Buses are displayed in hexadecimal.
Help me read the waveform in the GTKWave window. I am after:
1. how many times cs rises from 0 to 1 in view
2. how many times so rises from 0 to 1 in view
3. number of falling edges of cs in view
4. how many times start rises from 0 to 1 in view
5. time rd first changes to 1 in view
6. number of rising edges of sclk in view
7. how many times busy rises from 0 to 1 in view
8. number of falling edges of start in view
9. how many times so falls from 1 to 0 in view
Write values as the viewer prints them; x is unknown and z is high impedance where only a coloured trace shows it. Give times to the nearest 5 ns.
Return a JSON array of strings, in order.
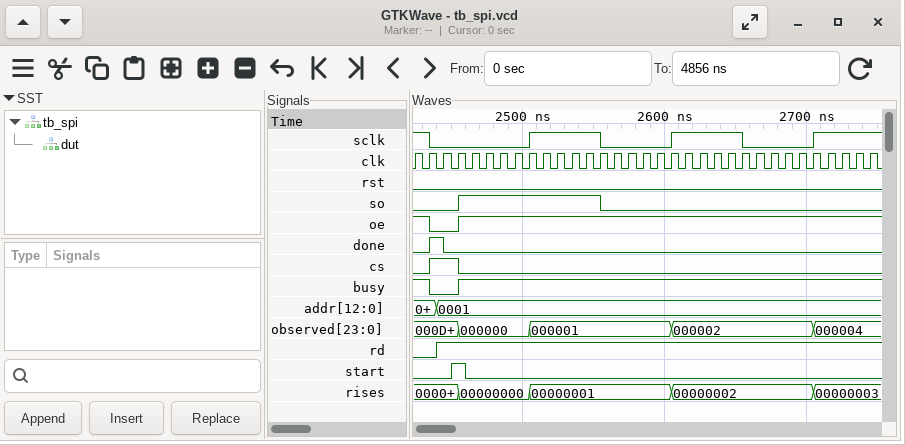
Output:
["1", "1", "1", "1", "2440 ns", "3", "1", "1", "1"]
